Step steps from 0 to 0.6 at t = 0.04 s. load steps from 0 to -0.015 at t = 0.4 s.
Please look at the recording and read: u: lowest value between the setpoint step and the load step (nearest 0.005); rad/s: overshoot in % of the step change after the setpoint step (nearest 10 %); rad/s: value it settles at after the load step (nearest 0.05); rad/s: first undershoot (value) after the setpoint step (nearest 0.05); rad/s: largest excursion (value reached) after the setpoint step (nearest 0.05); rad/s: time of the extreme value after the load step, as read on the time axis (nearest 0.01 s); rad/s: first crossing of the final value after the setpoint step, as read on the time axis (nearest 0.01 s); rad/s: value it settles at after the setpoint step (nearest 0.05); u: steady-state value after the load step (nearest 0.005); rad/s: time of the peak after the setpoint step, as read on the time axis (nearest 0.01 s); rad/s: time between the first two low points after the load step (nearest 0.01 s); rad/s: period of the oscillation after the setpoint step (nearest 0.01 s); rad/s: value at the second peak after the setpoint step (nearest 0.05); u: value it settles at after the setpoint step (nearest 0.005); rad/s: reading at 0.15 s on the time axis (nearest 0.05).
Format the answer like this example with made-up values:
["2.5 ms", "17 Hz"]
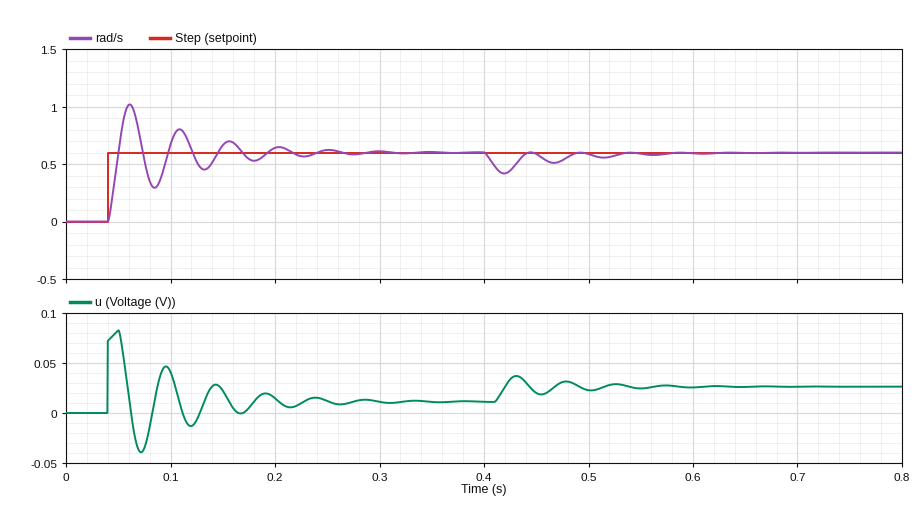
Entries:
["-0.040", "70 %", "0.60", "0.30", "1.00", "0.42 s", "0.05 s", "0.60", "0.025", "0.06 s", "0.05 s", "0.05 s", "0.80", "0.010", "0.65"]
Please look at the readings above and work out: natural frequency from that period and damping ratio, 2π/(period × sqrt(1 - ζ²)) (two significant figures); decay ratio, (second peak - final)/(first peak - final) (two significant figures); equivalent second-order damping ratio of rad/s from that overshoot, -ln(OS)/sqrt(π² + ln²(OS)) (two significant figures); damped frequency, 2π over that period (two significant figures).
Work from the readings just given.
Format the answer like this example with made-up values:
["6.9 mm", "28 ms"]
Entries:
["130 rad/s", "0.50", "0.11", "130 rad/s"]
